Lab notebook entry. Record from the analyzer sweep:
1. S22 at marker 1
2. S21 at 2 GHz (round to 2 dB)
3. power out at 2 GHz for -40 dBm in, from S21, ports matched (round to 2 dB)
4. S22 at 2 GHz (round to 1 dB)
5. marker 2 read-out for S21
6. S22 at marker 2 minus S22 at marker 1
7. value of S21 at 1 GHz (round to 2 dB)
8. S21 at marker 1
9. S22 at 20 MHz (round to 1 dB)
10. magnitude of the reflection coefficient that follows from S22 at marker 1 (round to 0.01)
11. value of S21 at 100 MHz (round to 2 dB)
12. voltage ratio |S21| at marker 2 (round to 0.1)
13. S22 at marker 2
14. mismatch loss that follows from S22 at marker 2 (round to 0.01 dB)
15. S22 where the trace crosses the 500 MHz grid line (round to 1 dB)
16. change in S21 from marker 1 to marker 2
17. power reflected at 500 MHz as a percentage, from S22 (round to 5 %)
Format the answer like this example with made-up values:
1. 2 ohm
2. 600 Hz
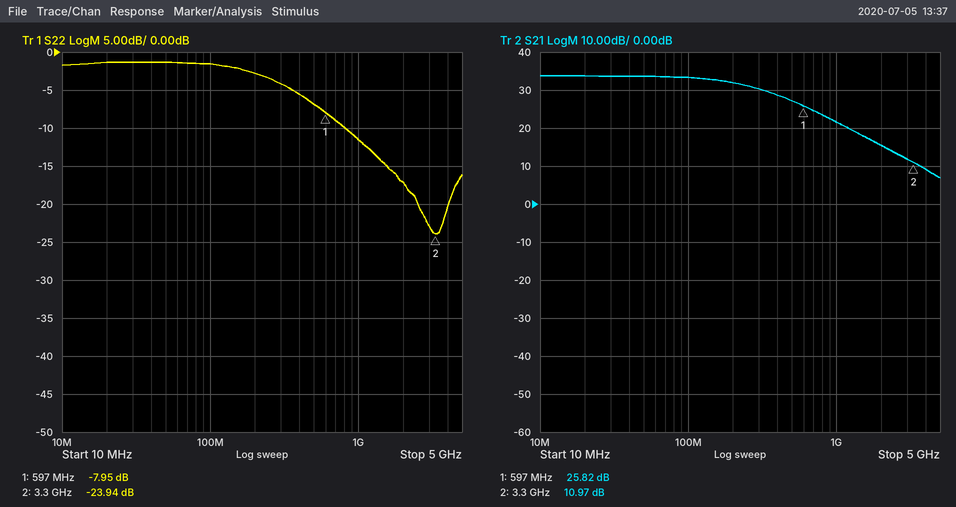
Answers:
1. -7.95 dB
2. 16 dB
3. -24 dBm
4. -17 dB
5. 10.97 dB
6. -15.99 dB
7. 22 dB
8. 25.82 dB
9. -1 dB
10. 0.40
11. 34 dB
12. 3.5
13. -23.94 dB
14. 0.02 dB
15. -7 dB
16. -14.85 dB
17. 20 %
